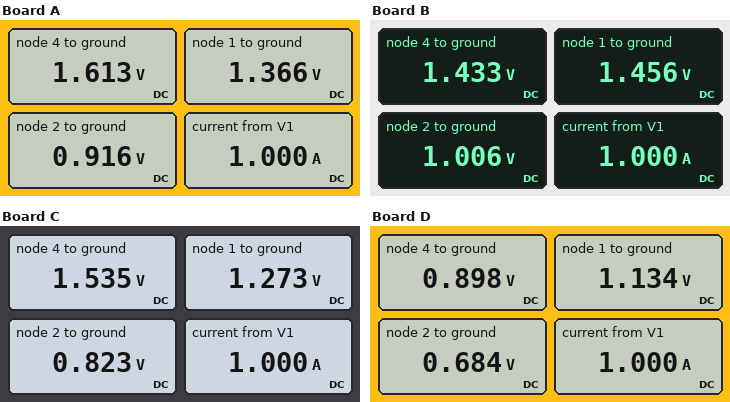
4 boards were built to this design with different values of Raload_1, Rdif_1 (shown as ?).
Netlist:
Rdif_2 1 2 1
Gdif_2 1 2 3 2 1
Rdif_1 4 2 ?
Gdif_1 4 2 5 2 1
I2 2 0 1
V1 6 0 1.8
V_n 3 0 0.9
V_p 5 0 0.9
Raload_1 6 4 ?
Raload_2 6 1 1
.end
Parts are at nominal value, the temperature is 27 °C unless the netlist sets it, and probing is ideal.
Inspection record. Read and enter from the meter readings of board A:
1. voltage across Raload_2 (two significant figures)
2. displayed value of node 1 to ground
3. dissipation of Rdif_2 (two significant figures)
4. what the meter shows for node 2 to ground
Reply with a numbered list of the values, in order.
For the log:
1. 430 mV
2. 1.366 V
3. 200 mW
4. 0.916 V
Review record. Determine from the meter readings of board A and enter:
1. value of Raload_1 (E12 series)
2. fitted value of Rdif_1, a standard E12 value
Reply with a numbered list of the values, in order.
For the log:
1. 0.33 Ω
2. 1.2 Ω
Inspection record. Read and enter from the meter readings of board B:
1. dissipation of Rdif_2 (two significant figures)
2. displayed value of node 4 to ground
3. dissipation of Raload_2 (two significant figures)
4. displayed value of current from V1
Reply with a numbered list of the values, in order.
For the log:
1. 200 mW
2. 1.433 V
3. 120 mW
4. 1.000 A
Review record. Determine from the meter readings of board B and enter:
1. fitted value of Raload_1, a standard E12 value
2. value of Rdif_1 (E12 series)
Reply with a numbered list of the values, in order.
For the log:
1. 0.56 Ω
2. 0.56 Ω
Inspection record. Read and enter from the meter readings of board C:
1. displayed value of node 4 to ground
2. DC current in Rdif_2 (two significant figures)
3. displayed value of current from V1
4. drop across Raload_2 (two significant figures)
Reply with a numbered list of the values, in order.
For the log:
1. 1.535 V
2. 450 mA
3. 1.000 A
4. 530 mV
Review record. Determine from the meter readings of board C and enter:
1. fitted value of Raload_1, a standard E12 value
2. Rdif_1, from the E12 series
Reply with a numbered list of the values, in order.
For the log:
1. 0.56 Ω
2. 1.8 Ω
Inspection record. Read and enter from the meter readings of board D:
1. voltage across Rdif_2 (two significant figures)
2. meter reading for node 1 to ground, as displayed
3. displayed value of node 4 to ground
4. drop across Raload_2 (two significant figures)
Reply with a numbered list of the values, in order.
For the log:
1. 450 mV
2. 1.134 V
3. 0.898 V
4. 670 mV
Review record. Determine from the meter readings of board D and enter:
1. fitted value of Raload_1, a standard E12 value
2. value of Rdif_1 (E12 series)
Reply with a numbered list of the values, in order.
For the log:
1. 2.7 Ω
2. 1.8 Ω
